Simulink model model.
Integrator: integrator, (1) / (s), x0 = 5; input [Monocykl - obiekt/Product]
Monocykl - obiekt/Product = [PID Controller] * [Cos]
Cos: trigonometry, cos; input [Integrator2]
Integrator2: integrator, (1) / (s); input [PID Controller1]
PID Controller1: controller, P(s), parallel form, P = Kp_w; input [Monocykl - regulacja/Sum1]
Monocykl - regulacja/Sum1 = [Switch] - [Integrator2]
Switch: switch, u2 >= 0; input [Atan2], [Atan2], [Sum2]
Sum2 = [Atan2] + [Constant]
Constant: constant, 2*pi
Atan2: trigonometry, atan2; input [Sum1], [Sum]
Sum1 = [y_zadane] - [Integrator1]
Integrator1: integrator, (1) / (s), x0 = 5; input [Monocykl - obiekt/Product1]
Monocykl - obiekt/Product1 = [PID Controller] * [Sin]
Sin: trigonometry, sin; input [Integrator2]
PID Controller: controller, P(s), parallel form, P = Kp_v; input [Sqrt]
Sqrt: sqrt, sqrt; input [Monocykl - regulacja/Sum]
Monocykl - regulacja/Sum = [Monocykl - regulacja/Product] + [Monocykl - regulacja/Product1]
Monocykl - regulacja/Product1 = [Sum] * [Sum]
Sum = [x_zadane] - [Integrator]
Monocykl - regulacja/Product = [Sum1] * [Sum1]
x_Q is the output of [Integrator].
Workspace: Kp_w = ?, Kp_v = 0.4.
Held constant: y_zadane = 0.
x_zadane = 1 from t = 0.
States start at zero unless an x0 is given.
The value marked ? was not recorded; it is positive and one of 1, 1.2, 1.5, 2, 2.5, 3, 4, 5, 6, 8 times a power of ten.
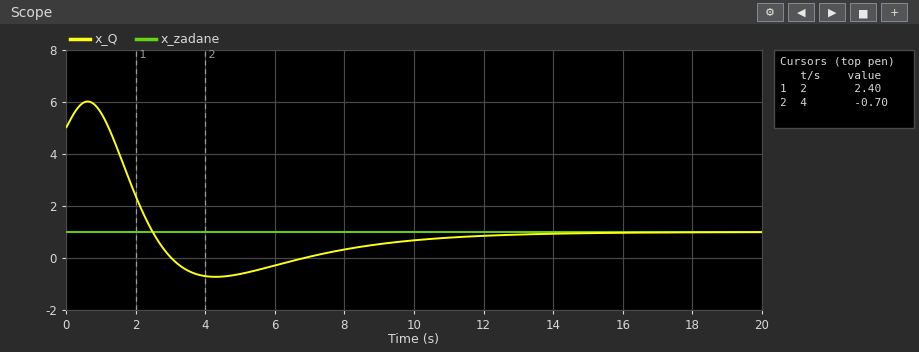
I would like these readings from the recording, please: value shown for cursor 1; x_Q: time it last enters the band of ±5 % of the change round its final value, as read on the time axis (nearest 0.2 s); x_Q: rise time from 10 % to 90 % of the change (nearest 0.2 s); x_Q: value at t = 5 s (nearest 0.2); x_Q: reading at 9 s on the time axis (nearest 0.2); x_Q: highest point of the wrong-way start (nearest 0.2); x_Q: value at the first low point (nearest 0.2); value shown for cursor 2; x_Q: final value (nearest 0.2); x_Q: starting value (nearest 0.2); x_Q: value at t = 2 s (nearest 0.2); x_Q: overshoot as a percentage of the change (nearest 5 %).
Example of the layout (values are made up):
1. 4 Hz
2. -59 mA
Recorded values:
1. 2.40
2. 11.2 s
3. 1.0 s
4. -0.6
5. 0.6
6. 6.0
7. -0.8
8. -0.70
9. 1.0
10. 5.0
11. 2.4
12. 45 %
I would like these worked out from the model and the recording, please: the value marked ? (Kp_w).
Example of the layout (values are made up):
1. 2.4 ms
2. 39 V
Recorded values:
1. 0.8
